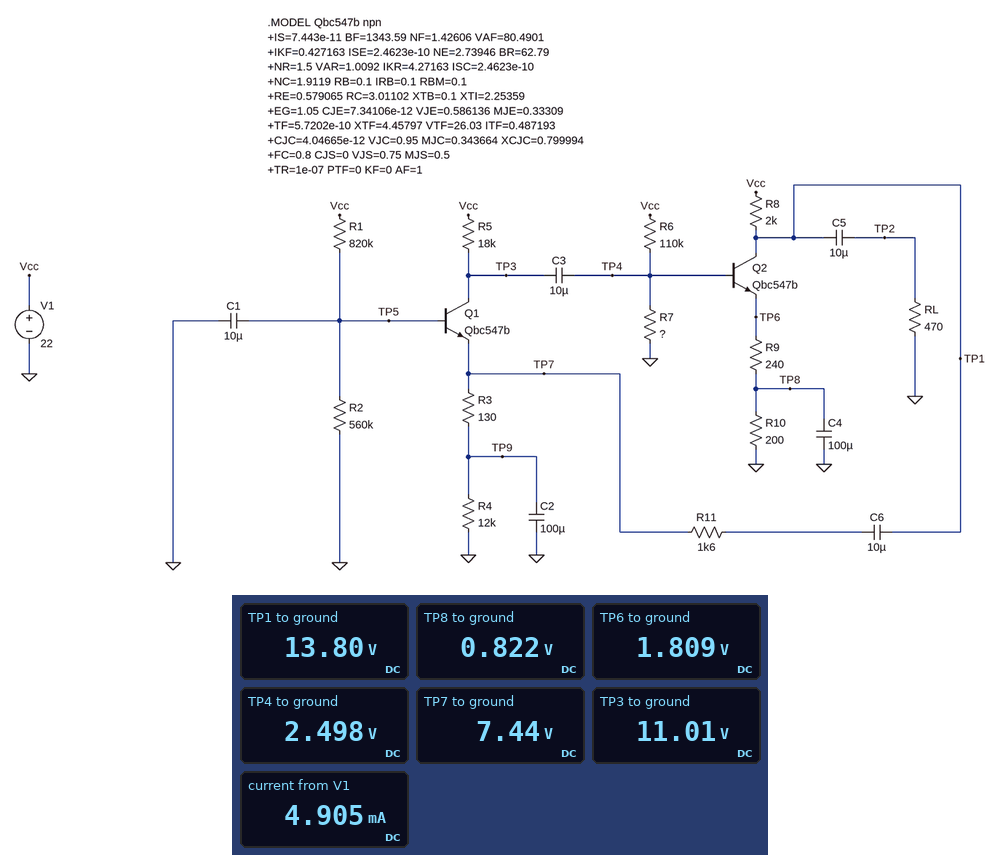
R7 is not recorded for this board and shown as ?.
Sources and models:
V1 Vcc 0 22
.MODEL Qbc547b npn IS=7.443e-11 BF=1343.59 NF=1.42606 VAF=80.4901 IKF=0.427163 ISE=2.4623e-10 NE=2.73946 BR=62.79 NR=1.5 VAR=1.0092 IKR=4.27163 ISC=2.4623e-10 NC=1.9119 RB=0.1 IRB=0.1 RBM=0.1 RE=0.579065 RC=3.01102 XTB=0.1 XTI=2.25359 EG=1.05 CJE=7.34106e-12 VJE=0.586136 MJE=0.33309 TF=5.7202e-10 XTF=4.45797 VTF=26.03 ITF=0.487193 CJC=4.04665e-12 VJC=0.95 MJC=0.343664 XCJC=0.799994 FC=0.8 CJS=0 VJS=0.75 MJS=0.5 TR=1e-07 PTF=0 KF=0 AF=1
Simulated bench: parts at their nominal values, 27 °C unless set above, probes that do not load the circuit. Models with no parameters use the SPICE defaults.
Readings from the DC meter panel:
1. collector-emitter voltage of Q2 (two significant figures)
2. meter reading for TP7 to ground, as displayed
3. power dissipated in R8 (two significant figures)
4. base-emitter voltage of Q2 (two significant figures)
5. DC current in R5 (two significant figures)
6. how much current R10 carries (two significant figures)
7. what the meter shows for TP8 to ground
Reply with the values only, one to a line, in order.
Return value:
12 V
7.44 V
34 mW
690 mV
610 µA
4.1 mA
0.822 V
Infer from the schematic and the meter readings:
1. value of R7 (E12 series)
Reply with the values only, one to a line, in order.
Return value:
15 kΩ
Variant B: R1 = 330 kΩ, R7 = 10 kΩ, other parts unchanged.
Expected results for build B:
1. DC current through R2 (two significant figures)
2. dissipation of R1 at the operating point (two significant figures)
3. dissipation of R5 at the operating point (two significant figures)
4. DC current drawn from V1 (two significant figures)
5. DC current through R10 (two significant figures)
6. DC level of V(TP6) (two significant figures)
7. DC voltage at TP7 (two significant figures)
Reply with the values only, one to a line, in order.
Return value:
17 µA
470 µW
9.3 mW
3.5 mA
2.5 mA
1.1 V
9.0 V
